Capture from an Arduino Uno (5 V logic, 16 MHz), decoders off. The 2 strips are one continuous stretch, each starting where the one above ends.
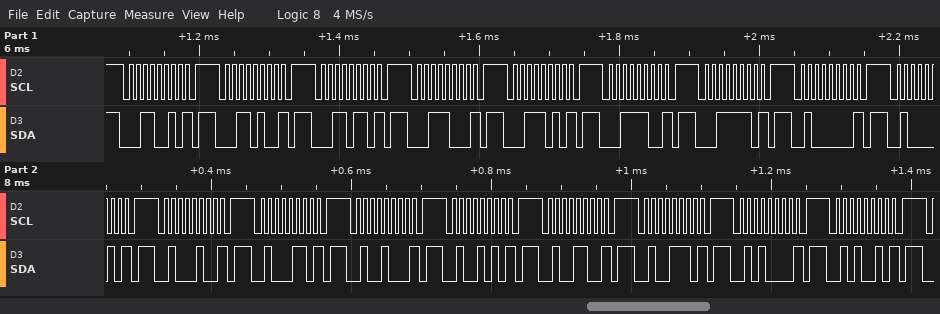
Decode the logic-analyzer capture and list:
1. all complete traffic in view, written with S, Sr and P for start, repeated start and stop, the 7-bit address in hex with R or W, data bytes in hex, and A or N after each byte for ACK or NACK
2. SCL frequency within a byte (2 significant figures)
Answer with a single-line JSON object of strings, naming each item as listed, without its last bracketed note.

{"all complete traffic in view, written with S, Sr and P for start, repeated start and stop, the 7-bit address in hex with R or W, data bytes in hex, and A or N after each byte for ACK or NACK": "S 19W N P S 1AW N P S 1BW N P S 1CW N P S 1DW N P S 1EW N P S 1FW N P S 20W N P S 21W N P S 22W N P S 23W N P S 24W N P S 25W N P S 26W N P S 27W N P S 28W N P S 29W N P", "SCL frequency within a byte": "100 kHz"}
